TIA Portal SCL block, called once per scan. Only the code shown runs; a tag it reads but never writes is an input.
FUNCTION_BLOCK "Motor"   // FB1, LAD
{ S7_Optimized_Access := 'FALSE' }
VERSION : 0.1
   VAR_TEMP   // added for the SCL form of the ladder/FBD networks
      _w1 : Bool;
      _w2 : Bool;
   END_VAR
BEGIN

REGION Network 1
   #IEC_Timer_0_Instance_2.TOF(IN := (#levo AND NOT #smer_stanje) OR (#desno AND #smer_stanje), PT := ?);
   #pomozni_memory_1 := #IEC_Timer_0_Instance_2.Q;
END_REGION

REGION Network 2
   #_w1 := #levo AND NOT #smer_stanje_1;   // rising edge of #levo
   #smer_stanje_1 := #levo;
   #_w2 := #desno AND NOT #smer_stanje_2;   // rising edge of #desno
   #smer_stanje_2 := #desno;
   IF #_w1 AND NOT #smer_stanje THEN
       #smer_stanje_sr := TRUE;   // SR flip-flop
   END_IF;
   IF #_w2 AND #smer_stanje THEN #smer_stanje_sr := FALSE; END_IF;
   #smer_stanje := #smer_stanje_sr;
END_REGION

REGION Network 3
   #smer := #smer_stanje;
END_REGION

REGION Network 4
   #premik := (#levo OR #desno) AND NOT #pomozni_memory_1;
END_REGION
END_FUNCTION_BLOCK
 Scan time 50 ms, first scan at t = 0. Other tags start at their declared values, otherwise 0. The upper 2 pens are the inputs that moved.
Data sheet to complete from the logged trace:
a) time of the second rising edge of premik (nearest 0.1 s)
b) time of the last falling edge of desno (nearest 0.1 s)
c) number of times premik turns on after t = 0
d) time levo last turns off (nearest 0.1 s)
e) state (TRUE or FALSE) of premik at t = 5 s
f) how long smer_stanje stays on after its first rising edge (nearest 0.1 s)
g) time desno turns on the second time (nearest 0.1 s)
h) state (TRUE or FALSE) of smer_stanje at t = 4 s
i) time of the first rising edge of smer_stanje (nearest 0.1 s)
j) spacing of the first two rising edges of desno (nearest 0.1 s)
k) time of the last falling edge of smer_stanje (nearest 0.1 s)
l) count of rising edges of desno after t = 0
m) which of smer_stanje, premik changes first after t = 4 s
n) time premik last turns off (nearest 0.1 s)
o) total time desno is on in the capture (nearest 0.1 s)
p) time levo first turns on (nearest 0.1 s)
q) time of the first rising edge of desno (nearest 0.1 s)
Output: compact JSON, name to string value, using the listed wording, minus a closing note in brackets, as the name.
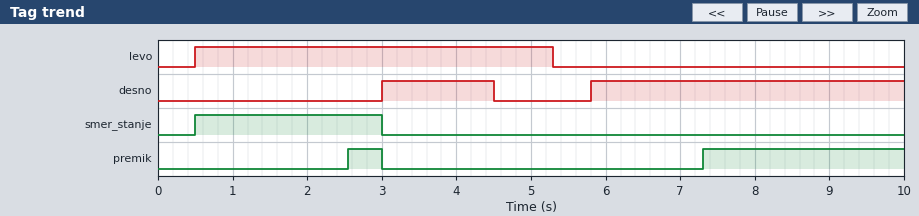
{"time of the second rising edge of premik": "7.3 s", "time of the last falling edge of desno": "4.5 s", "number of times premik turns on after t = 0": "2", "time levo last turns off": "5.3 s", "state (TRUE or FALSE) of premik at t = 5 s": "FALSE", "how long smer_stanje stays on after its first rising edge": "2.5 s", "time desno turns on the second time": "5.8 s", "state (TRUE or FALSE) of smer_stanje at t = 4 s": "FALSE", "time of the first rising edge of smer_stanje": "0.5 s", "spacing of the first two rising edges of desno": "2.8 s", "time of the last falling edge of smer_stanje": "3.0 s", "count of rising edges of desno after t = 0": "2", "which of smer_stanje, premik changes first after t = 4 s": "premik", "time premik last turns off": "3.0 s", "total time desno is on in the capture": "5.7 s", "time levo first turns on": "0.5 s", "time of the first rising edge of desno": "3.0 s"}
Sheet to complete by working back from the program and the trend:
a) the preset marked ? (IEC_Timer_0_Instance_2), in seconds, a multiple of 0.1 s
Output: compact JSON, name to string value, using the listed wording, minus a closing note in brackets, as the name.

{"the preset marked ? (IEC_Timer_0_Instance_2), in seconds, a multiple of 0.1 s": "2.0 s"}
